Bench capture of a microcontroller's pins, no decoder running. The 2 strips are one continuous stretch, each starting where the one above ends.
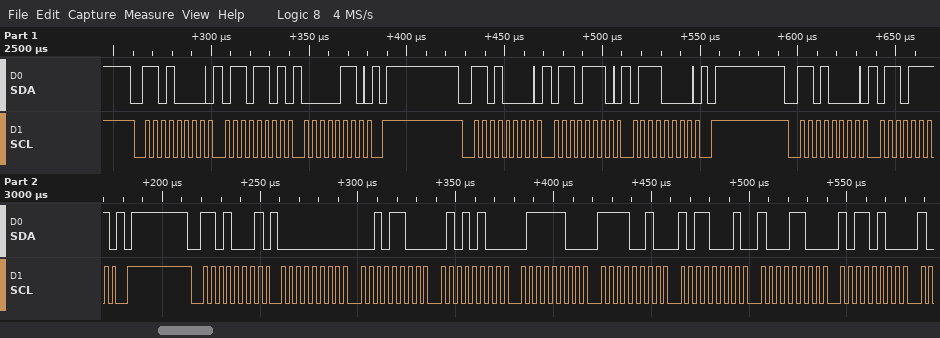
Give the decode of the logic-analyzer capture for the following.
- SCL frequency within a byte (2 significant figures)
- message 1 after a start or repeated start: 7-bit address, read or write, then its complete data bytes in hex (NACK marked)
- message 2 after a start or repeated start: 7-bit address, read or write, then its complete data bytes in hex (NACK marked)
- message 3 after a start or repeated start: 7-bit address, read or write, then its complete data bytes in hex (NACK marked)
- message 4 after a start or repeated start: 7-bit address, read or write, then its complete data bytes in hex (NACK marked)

250 kHz
0x68 write: 6D 06
0x68 write: 6E 70
0x68 write: 6F
0x68 read: 00 2C 54 7C F2 B1 8C B4
